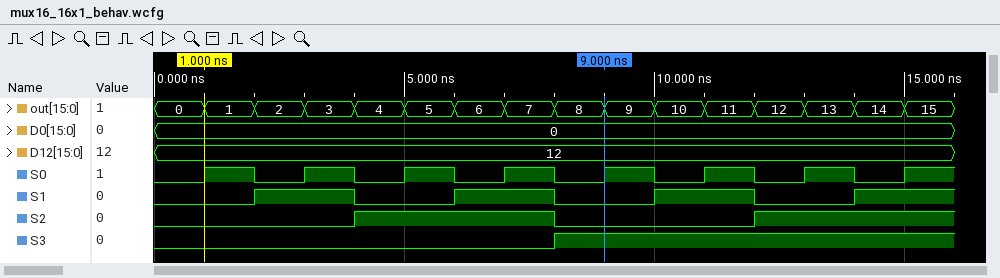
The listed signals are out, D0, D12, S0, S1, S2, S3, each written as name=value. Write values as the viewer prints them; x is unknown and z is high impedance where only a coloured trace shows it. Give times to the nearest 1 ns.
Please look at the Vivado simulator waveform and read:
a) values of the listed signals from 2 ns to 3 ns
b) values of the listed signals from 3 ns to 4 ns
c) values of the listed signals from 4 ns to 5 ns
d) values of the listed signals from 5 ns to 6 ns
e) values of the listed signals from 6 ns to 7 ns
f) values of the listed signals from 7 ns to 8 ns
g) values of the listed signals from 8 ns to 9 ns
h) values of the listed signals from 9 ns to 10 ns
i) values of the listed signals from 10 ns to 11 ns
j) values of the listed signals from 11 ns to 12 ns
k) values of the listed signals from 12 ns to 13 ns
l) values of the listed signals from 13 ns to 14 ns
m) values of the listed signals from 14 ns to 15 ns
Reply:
out=2, D0=0, D12=12, S0=0, S1=1, S2=0, S3=0
out=3, D0=0, D12=12, S0=1, S1=1, S2=0, S3=0
out=4, D0=0, D12=12, S0=0, S1=0, S2=1, S3=0
out=5, D0=0, D12=12, S0=1, S1=0, S2=1, S3=0
out=6, D0=0, D12=12, S0=0, S1=1, S2=1, S3=0
out=7, D0=0, D12=12, S0=1, S1=1, S2=1, S3=0
out=8, D0=0, D12=12, S0=0, S1=0, S2=0, S3=1
out=9, D0=0, D12=12, S0=1, S1=0, S2=0, S3=1
out=10, D0=0, D12=12, S0=0, S1=1, S2=0, S3=1
out=11, D0=0, D12=12, S0=1, S1=1, S2=0, S3=1
out=12, D0=0, D12=12, S0=0, S1=0, S2=1, S3=1
out=13, D0=0, D12=12, S0=1, S1=0, S2=1, S3=1
out=14, D0=0, D12=12, S0=0, S1=1, S2=1, S3=1
